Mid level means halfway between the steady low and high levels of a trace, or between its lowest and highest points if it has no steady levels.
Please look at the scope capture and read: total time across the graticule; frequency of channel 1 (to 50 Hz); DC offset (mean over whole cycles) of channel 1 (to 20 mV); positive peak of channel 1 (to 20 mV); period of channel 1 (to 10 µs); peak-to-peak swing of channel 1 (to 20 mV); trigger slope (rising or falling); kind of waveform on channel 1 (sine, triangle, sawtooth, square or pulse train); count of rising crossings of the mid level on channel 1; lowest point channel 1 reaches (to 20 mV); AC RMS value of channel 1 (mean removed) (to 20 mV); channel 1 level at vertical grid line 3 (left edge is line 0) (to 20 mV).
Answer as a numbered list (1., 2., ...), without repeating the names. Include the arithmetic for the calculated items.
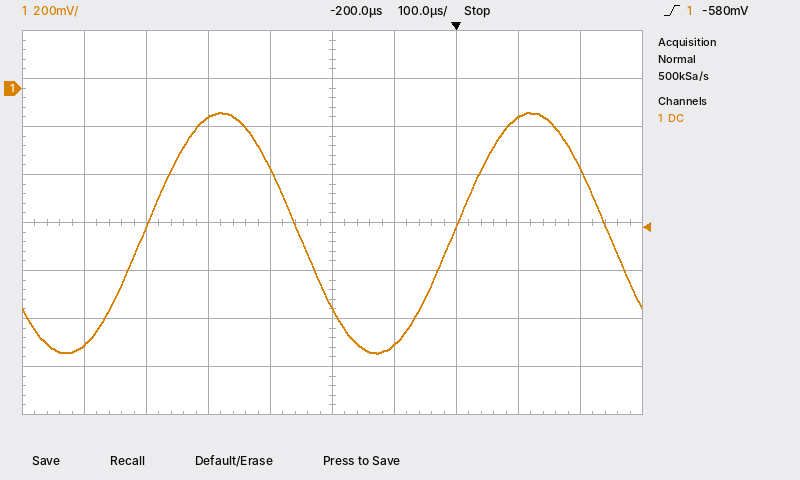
1. 1 ms
2. 1 / 500 µs ≈ 2.00 kHz
3. (-100 mV + (-1.10 V)) / 2 ≈ -600 mV
4. -100 mV
5. 500 µs
6. -100 mV − (-1.10 V) = 1.00 V
7. rising
8. sine
9. 2
10. -1.10 V
11. 1.00 V / (2√2) ≈ 354 mV, so 360 mV to the nearest 20 mV
12. -120 mV
